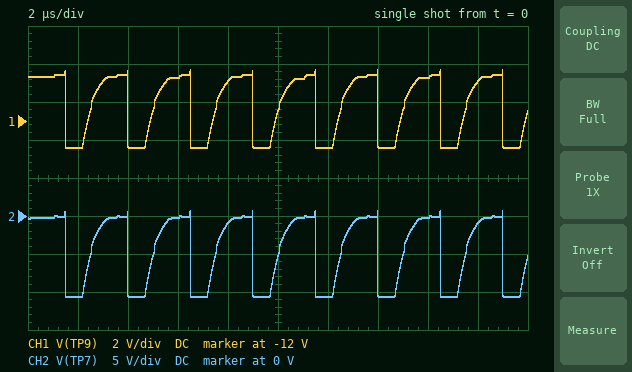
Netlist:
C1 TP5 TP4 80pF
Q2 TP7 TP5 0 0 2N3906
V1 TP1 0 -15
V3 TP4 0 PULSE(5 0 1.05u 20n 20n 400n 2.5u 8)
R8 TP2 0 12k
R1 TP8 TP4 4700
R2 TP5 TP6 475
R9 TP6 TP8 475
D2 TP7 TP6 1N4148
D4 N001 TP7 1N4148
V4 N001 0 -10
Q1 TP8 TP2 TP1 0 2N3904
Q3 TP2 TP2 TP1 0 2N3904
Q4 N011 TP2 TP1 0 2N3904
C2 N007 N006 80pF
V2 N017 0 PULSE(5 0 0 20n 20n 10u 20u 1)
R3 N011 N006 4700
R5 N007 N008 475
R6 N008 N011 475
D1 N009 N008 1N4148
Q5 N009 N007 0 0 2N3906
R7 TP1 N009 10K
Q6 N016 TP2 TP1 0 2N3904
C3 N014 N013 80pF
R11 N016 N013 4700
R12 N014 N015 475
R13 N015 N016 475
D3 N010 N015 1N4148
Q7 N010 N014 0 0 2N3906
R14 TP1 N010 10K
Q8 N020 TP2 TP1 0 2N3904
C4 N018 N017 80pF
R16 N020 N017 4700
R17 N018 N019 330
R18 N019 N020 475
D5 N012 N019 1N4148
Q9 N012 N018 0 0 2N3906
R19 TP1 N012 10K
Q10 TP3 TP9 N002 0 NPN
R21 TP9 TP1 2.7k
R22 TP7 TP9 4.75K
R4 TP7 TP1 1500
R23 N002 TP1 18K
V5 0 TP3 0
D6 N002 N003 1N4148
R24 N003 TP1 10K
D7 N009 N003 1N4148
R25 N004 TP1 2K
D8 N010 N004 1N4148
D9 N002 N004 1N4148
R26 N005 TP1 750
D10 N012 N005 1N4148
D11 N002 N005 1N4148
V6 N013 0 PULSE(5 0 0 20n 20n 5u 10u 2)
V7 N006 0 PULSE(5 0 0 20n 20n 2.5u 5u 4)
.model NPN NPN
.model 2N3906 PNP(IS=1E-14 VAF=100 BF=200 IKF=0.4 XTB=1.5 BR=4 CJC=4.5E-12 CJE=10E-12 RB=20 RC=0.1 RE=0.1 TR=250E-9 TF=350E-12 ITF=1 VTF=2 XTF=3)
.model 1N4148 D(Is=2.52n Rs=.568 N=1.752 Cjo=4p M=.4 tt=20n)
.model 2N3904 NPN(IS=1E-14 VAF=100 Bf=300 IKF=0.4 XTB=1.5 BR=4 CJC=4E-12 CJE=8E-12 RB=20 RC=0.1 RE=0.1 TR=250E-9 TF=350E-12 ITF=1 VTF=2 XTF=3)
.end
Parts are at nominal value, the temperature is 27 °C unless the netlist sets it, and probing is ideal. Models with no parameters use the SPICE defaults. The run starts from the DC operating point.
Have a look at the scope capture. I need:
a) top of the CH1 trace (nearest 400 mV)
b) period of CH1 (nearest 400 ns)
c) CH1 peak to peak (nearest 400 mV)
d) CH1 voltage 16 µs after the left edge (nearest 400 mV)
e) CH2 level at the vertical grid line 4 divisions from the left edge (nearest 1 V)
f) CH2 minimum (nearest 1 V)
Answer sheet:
-9.2 V
2.4 µs
4.0 V
-9.6 V
-1 V
-11 V
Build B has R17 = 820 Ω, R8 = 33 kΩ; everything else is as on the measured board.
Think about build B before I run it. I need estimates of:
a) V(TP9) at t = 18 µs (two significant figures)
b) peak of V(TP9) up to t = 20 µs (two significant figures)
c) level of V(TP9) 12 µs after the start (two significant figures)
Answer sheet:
-13 V
-9.6 V
-13 V
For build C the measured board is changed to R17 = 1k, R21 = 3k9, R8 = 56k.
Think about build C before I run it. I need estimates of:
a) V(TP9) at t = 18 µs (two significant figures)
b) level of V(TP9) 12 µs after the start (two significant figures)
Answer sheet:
-13 V
-13 V
